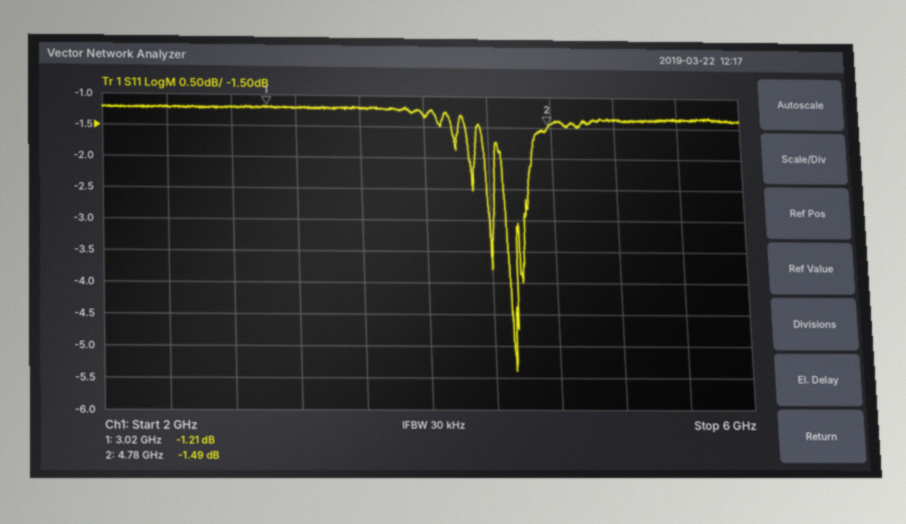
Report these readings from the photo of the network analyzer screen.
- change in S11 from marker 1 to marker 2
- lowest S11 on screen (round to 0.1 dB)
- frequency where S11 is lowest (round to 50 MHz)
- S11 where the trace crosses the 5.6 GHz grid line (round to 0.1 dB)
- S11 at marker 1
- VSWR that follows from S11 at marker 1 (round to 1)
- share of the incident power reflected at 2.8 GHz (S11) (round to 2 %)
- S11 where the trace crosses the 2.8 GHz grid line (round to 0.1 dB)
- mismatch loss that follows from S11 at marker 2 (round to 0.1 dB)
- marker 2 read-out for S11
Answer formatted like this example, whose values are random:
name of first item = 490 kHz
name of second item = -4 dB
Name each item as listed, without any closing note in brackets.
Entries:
change in S11 from marker 1 to marker 2 = -0.28 dB
lowest S11 on screen = -5.4 dB
frequency where S11 is lowest = 4.55 GHz
S11 where the trace crosses the 5.6 GHz grid line = -1.4 dB
S11 at marker 1 = -1.21 dB
VSWR that follows from S11 at marker 1 = 14
share of the incident power reflected at 2.8 GHz (S11) = 76 %
S11 where the trace crosses the 2.8 GHz grid line = -1.2 dB
mismatch loss that follows from S11 at marker 2 = 5.4 dB
marker 2 read-out for S11 = -1.49 dB
